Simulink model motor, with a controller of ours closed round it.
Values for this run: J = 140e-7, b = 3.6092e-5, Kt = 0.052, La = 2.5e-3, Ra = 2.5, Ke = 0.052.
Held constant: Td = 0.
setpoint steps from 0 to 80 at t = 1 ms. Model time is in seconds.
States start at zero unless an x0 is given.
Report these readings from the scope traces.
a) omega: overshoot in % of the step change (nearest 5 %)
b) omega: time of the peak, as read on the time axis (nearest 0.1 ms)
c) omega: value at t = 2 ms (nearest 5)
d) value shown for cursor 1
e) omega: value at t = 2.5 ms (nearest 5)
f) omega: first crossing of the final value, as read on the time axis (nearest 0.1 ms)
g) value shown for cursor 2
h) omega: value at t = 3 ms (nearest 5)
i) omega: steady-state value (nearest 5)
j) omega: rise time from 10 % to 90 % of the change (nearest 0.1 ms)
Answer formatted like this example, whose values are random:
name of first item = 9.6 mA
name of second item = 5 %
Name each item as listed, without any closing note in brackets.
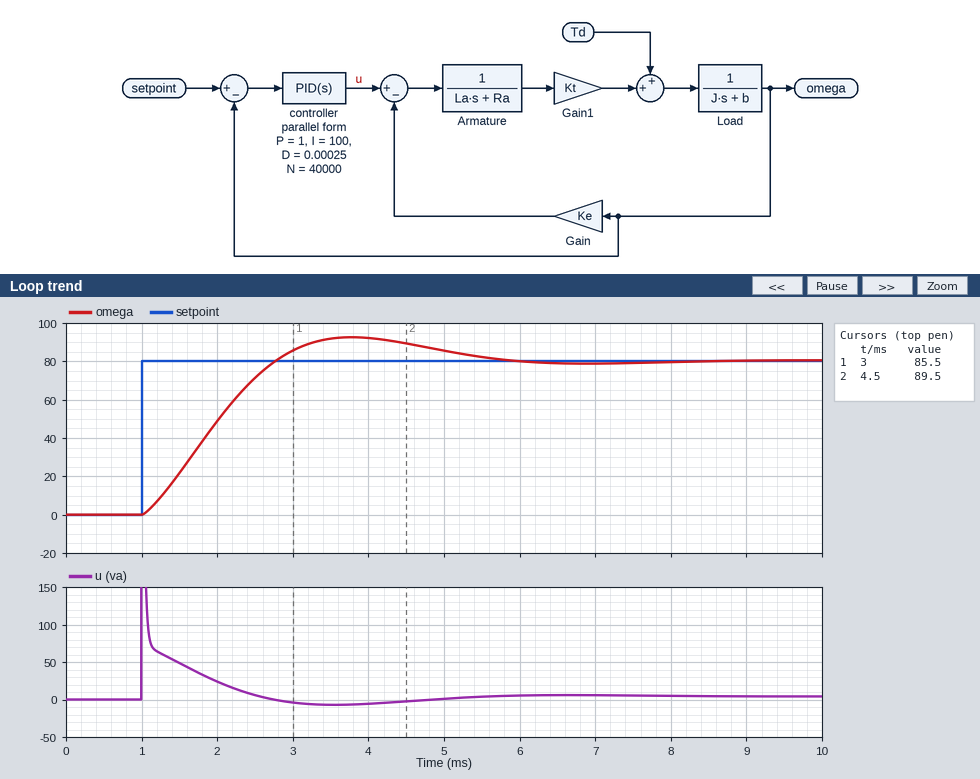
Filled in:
omega: overshoot in % of the step change = 15 %
omega: time of the peak, as read on the time axis = 3.8 ms
omega: value at t = 2 ms = 50
value shown for cursor 1 = 85.5
omega: value at t = 2.5 ms = 70
omega: first crossing of the final value, as read on the time axis = 2.8 ms
value shown for cursor 2 = 89.5
omega: value at t = 3 ms = 85
omega: steady-state value = 80
omega: rise time from 10 % to 90 % of the change = 1.3 ms
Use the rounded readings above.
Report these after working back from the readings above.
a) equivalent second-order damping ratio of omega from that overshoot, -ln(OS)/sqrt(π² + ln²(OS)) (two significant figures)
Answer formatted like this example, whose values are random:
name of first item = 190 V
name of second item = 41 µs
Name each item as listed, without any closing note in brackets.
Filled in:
equivalent second-order damping ratio of omega from that overshoot, -ln(OS)/sqrt(π² + ln²(OS)) = 0.52
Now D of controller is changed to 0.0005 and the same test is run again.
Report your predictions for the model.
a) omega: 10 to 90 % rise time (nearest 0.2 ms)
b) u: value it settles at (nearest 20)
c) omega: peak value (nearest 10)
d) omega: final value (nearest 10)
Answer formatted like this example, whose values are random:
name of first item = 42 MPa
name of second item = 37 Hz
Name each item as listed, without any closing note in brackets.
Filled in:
omega: 10 to 90 % rise time = 1.4 ms
u: value it settles at = 0
omega: peak value = 90
omega: final value = 80
